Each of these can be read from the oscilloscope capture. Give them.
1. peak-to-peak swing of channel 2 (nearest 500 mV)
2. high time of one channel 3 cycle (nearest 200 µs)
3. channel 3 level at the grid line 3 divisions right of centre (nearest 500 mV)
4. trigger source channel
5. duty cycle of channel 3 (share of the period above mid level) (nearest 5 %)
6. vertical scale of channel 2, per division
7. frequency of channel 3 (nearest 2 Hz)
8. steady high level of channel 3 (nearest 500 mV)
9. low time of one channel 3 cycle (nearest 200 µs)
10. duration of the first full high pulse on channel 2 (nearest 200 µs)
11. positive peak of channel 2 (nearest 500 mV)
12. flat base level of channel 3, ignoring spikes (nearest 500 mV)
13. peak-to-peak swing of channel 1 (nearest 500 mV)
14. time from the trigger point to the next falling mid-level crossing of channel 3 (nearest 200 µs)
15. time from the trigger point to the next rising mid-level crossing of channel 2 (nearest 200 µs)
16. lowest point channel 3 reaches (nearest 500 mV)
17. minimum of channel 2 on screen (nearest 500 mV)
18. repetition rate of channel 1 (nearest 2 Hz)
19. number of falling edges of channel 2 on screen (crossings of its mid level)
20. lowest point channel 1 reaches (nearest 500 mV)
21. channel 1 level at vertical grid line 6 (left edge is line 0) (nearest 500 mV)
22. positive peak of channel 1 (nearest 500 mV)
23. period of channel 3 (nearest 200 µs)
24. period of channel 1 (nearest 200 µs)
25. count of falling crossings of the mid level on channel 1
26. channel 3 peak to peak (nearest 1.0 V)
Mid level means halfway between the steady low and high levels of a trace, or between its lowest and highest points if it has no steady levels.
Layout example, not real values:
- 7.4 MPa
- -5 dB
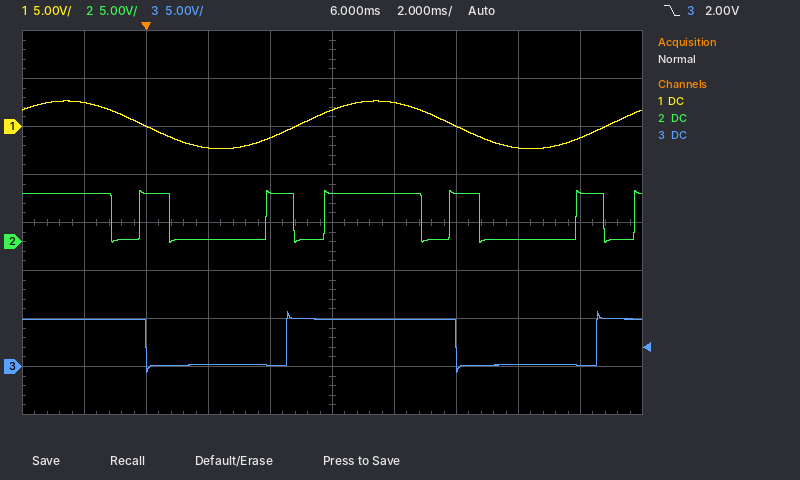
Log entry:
- 5.5 V
- 5.4 ms
- 0.0 V
- channel 3
- 55 %
- 5 V
- 100 Hz
- 5.0 V
- 4.6 ms
- 1.0 ms
- 5.5 V
- 0.0 V
- 5.0 V
- 10.0 ms
- 3.8 ms
- -500 mV
- 0.0 V
- 100 Hz
- 6
- -2.5 V
- 2.5 V
- 2.5 V
- 10.0 ms
- 10.0 ms
- 2
- 6.0 V
